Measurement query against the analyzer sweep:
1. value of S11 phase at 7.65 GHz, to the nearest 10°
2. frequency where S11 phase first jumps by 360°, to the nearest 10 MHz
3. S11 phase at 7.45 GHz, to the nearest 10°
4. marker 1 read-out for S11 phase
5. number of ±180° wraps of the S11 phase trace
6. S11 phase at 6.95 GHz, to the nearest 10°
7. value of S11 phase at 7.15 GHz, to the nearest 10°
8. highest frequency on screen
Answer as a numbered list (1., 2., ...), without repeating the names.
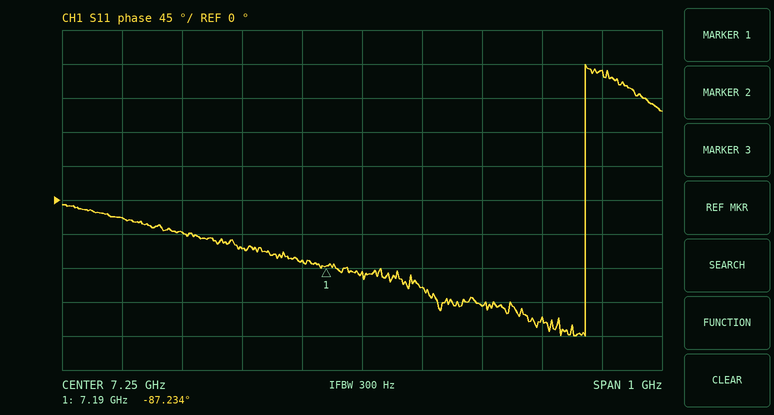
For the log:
1. 170°
2. 7.62 GHz
3. -140°
4. -87.234°
5. 1
6. -40°
7. -80°
8. 7.75 GHz
